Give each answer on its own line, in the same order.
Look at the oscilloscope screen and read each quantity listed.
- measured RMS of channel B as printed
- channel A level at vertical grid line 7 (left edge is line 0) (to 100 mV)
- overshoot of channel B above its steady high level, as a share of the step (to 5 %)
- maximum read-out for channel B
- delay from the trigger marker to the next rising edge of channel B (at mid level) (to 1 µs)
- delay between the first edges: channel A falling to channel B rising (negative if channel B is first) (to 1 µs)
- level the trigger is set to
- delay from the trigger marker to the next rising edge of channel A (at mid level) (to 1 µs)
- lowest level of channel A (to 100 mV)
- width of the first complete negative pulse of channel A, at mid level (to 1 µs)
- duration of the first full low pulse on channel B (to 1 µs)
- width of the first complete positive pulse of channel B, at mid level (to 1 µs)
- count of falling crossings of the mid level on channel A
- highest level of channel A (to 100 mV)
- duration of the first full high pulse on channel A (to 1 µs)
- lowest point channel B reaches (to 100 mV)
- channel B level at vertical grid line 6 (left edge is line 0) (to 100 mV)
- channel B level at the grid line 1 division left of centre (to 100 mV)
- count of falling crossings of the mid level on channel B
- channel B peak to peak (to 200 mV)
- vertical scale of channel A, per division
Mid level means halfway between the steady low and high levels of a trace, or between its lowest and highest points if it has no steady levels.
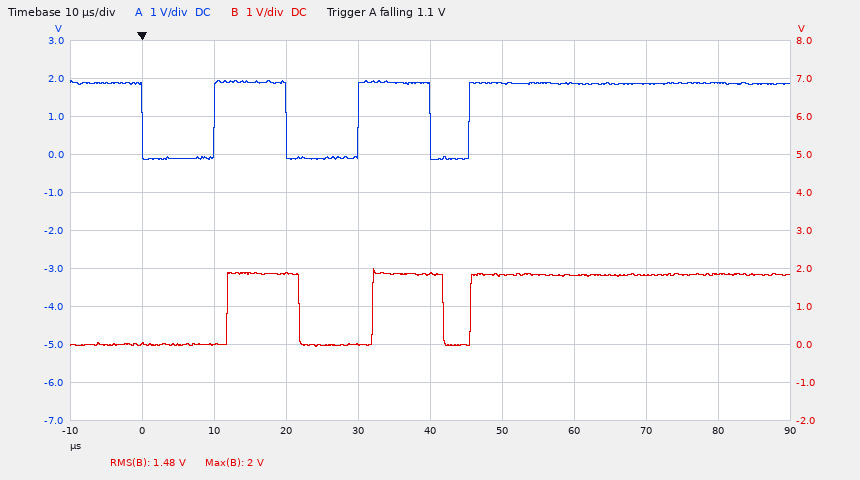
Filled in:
1.48 V
1.9 V
10 %
2 V
12 µs
+12 µs
1.1 V
10 µs
-100 mV
10 µs
10 µs
10 µs
3
1.9 V
10 µs
-100 mV
1.8 V
0.0 V
2
2.0 V
1 V
